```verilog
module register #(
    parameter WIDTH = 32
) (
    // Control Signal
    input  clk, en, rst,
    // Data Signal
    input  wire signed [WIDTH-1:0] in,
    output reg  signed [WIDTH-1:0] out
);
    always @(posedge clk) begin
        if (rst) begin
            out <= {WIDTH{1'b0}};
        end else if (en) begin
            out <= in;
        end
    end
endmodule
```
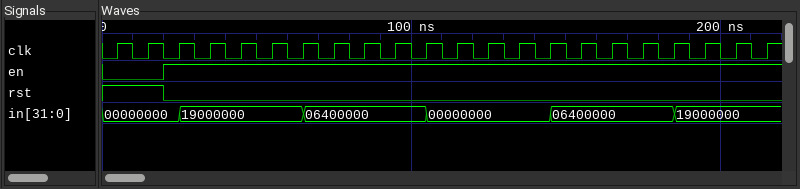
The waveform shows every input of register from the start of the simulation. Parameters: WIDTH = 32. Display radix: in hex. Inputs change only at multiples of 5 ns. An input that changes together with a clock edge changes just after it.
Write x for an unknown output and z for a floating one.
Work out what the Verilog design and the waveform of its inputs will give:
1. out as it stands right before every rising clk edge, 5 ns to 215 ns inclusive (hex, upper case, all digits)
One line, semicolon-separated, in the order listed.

x, 00000000, 00000000, 00000000, 19000000, 19000000, 19000000, 19000000, 06400000, 06400000, 06400000, 06400000, 00000000, 00000000, 00000000, 00000000, 06400000, 06400000, 06400000, 06400000, 19000000, 19000000
